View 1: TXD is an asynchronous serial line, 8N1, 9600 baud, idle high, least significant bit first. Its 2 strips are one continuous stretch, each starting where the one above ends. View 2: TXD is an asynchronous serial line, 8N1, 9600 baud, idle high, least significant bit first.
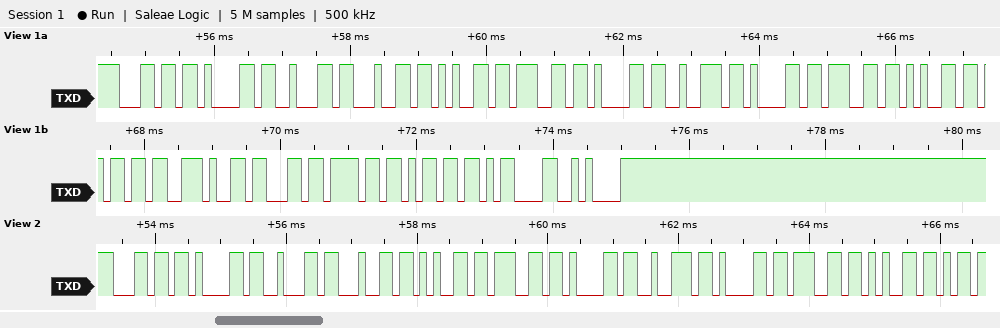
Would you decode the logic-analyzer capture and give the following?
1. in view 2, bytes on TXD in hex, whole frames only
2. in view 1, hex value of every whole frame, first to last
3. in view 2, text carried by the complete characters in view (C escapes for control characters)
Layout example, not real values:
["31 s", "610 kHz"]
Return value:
["6C 61 62 64 65 67 61 72 61 67 65", "0x6C 0x61 0x62 0x64 0x65 0x67 0x61 0x72 0x61 0x67 0x65 0x6D 0x2E 0x63 0x6F 0x6D 0x0D 0x0A", "\"labdegarage\""]
